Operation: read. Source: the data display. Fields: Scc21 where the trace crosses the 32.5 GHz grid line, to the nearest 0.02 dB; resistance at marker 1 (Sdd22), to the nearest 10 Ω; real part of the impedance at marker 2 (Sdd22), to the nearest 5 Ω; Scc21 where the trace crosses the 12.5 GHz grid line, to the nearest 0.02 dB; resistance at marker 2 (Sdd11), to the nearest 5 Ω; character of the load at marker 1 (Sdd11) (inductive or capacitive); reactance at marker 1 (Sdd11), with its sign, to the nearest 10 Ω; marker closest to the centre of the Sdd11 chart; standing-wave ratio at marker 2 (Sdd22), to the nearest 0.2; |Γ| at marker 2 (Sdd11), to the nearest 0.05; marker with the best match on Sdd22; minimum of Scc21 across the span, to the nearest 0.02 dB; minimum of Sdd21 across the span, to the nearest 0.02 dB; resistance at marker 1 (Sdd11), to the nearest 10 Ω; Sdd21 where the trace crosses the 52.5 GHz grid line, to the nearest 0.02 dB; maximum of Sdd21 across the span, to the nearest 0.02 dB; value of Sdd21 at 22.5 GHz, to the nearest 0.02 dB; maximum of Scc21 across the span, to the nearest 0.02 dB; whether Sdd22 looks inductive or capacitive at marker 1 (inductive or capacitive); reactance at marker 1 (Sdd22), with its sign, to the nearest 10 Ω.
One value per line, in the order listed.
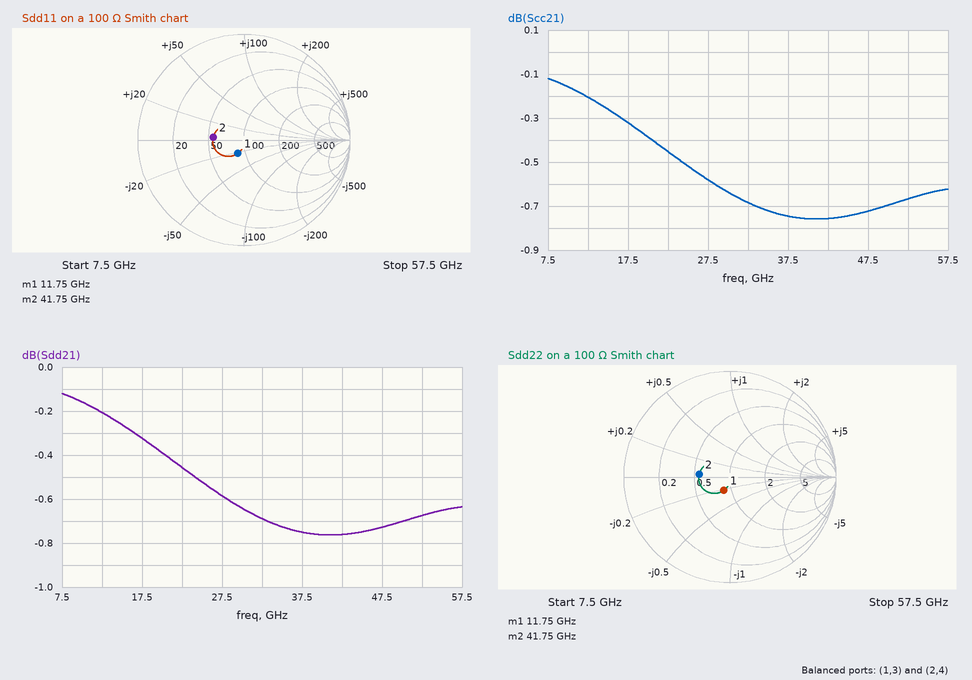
-0.68 dB
90 Ω
55 Ω
-0.20 dB
55 Ω
capacitive
-20 Ω
marker 1
1.8
0.30
marker 1
-0.76 dB
-0.76 dB
90 Ω
-0.68 dB
-0.12 dB
-0.46 dB
-0.12 dB
capacitive
-20 Ω
